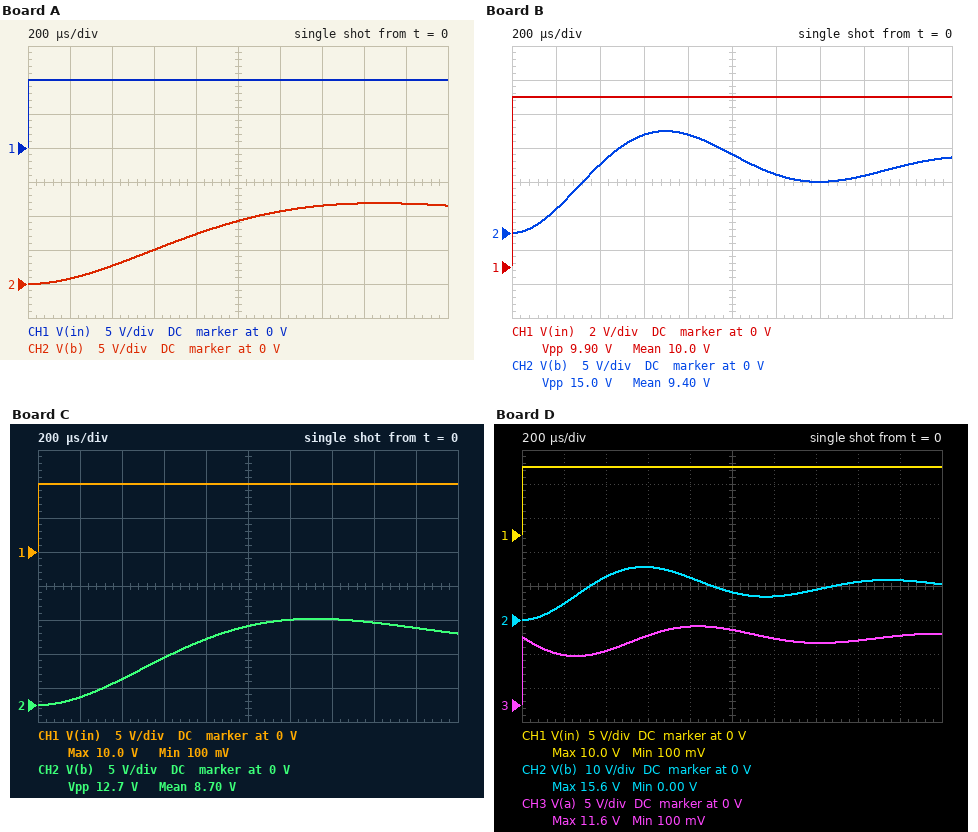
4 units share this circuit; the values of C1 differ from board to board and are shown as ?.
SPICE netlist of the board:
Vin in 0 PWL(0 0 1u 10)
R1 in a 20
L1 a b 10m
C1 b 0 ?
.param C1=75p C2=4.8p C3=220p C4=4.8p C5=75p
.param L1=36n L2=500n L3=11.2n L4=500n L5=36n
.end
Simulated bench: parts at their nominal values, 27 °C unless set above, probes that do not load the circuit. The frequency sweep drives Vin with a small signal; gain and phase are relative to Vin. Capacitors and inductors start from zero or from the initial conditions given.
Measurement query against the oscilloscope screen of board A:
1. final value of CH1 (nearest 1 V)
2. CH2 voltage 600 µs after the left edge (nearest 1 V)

10 V
5 V
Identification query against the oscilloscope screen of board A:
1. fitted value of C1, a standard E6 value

22 µF
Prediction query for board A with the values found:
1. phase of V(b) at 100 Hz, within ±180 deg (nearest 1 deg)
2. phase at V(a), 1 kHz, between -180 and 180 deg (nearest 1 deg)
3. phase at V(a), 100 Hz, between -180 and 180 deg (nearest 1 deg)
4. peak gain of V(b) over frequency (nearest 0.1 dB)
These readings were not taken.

-17 deg
20 deg
-17 deg
1.6 dB
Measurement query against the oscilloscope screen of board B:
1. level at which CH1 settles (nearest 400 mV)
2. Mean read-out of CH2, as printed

10.0 V
9.40 V
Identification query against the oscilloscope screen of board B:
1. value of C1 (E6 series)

4.7 µF
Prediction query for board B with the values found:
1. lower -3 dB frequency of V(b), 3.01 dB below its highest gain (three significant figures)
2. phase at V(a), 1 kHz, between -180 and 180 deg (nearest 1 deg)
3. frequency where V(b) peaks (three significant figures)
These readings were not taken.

510 Hz
35 deg
699 Hz
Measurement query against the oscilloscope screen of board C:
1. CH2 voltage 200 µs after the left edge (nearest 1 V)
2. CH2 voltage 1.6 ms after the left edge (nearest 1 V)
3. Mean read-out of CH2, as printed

1 V
12 V
8.70 V
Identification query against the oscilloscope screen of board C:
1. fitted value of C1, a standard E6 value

15 µF
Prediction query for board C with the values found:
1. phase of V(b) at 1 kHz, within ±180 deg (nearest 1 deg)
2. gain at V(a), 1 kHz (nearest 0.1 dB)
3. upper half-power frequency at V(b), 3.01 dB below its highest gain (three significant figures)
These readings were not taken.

-159 deg
-0.6 dB
489 Hz
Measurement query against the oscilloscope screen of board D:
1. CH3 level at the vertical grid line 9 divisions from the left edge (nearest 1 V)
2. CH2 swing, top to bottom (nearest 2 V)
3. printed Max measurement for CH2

10 V
16 V
15.6 V
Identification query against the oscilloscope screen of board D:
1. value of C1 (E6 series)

3.3 µF
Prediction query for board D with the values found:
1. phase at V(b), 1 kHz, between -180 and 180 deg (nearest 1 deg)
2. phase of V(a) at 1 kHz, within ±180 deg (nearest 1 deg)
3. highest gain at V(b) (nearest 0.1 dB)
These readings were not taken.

-126 deg
54 deg
8.9 dB
